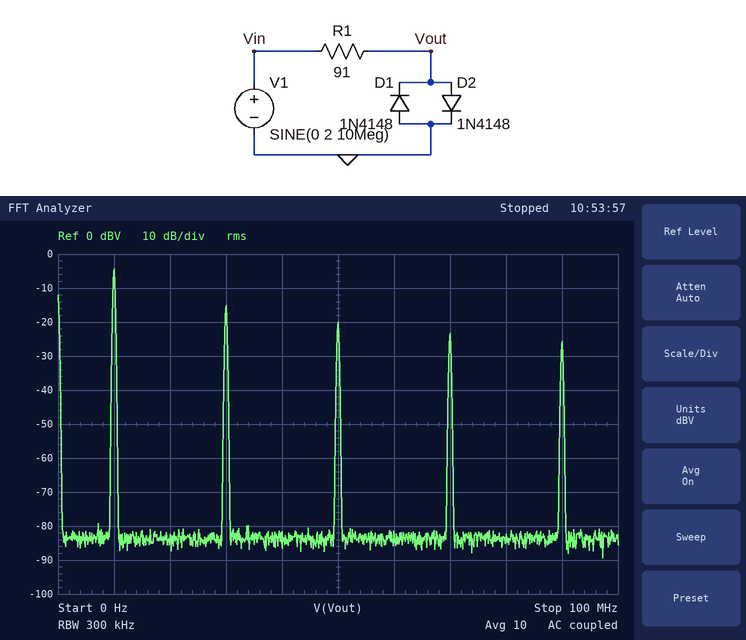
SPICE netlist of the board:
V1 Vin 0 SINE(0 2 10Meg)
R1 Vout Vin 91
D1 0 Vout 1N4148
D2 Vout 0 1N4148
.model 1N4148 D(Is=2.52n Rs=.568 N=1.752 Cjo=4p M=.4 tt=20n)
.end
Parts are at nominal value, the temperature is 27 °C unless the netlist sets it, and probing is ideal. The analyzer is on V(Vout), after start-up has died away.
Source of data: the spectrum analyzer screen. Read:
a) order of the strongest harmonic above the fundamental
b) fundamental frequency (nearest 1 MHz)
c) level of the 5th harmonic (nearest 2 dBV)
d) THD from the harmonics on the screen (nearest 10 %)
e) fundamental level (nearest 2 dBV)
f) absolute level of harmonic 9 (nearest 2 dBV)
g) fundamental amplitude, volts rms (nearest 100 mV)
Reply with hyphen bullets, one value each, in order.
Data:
- 3
- 10 MHz
- -20 dBV
- 40 %
- -4 dBV
- -26 dBV
- 600 mV
